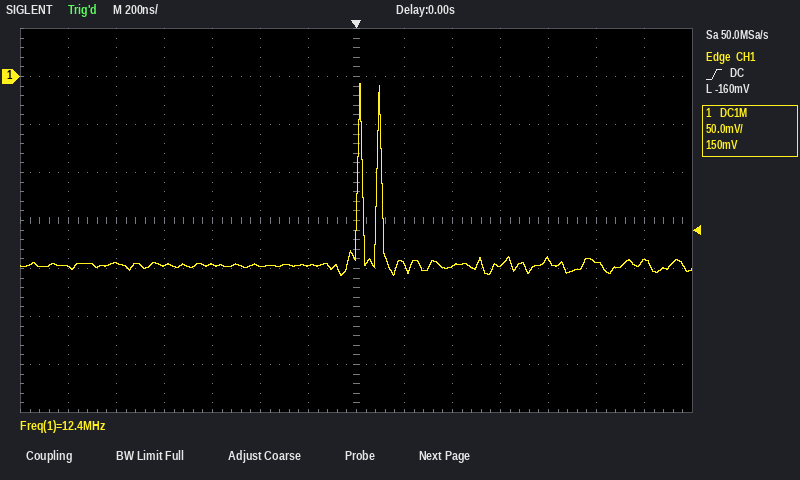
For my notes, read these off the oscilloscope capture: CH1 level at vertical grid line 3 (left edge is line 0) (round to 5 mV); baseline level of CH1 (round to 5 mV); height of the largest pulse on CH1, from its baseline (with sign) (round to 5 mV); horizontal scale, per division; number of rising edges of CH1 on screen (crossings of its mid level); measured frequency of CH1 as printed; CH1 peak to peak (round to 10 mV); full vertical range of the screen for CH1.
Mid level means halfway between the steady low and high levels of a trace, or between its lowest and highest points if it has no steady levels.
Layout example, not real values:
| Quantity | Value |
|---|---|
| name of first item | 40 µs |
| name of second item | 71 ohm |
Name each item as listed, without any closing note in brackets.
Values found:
| Quantity | Value |
|---|---|
| CH1 level at vertical grid line 3 (left edge is line 0) | -195 mV |
| baseline level of CH1 | -195 mV |
| height of the largest pulse on CH1, from its baseline (with sign) | +190 mV |
| horizontal scale, per division | 200 ns |
| number of rising edges of CH1 on screen | 2 |
| measured frequency of CH1 as printed | 12.4 MHz |
| CH1 peak to peak | 200 mV |
| full vertical range of the screen for CH1 | 400 mV |
